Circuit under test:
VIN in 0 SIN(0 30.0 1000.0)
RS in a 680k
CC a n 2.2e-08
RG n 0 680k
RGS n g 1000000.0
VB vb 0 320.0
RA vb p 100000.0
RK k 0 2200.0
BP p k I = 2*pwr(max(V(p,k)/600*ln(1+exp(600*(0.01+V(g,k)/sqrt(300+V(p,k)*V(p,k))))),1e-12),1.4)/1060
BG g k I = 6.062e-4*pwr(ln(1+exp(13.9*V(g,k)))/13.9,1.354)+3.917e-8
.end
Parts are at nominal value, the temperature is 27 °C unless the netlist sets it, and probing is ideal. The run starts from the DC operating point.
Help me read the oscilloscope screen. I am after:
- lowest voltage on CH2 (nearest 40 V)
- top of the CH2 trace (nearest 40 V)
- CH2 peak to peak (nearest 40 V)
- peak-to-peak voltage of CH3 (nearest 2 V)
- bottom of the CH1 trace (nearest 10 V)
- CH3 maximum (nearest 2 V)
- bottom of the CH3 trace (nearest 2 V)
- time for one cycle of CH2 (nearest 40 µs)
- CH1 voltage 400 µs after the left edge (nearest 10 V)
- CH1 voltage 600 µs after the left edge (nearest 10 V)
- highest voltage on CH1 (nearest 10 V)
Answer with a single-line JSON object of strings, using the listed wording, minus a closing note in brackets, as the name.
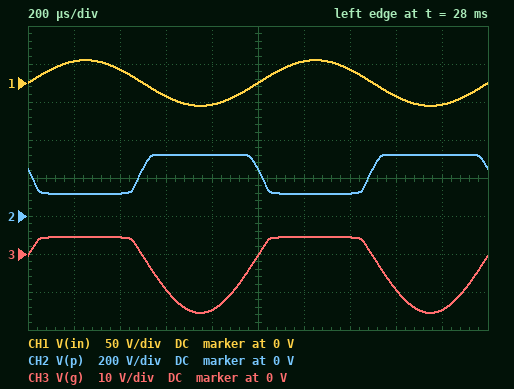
{"lowest voltage on CH2": "120 V", "top of the CH2 trace": "320 V", "CH2 peak to peak": "200 V", "peak-to-peak voltage of CH3": "20 V", "bottom of the CH1 trace": "-30 V", "CH3 maximum": "4 V", "bottom of the CH3 trace": "-16 V", "time for one cycle of CH2": "1.00 ms", "CH1 voltage 400 µs after the left edge": "20 V", "CH1 voltage 600 µs after the left edge": "-20 V", "highest voltage on CH1": "30 V"}
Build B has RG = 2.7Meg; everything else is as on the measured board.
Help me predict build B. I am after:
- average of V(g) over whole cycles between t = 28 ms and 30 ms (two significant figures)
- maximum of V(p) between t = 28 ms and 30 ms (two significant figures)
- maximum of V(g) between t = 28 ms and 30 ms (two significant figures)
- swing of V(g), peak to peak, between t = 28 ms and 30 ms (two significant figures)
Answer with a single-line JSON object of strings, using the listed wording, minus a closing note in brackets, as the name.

{"average of V(g) over whole cycles between t = 28 ms and 30 ms": "-6.9 V", "maximum of V(p) between t = 28 ms and 30 ms": "320 V", "maximum of V(g) between t = 28 ms and 30 ms": "4.6 V", "swing of V(g), peak to peak, between t = 28 ms and 30 ms": "31 V"}
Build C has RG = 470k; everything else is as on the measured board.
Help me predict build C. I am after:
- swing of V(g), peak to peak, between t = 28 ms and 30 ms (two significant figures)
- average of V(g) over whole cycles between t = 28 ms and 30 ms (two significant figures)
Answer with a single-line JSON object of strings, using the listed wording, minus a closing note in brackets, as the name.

{"swing of V(g), peak to peak, between t = 28 ms and 30 ms": "17 V", "average of V(g) over whole cycles between t = 28 ms and 30 ms": "-2.1 V"}
